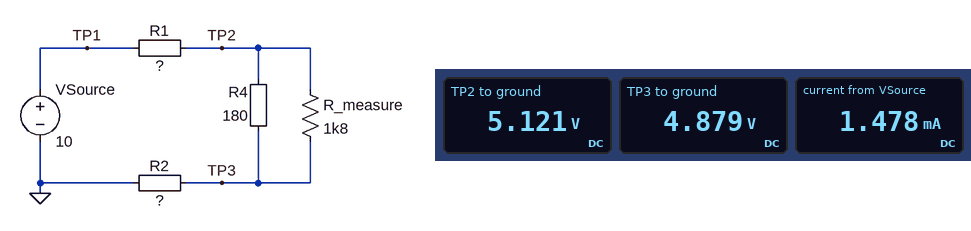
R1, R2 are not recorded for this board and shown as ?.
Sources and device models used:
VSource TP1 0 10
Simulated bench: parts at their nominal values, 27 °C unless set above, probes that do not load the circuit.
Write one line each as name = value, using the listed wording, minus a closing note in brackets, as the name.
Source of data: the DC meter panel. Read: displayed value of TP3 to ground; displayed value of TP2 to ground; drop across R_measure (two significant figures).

displayed value of TP3 to ground = 4.879 V
displayed value of TP2 to ground = 5.121 V
drop across R_measure = 240 mV
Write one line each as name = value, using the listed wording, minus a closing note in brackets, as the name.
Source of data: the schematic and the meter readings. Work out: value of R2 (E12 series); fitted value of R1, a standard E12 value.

value of R2 = 3.3 kΩ
fitted value of R1, a standard E12 value = 3.3 kΩ
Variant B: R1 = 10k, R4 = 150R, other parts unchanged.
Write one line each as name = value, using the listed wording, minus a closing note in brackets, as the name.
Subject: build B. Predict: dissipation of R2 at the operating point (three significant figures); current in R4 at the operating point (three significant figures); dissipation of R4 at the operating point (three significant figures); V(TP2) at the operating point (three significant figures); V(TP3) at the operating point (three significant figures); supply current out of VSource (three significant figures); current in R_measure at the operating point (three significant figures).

dissipation of R2 at the operating point = 1.83 mW
current in R4 at the operating point = 687 µA
dissipation of R4 at the operating point = 70.8 µW
V(TP2) at the operating point = 2.56 V
V(TP3) at the operating point = 2.46 V
supply current out of VSource = 744 µA
current in R_measure at the operating point = 57.2 µA
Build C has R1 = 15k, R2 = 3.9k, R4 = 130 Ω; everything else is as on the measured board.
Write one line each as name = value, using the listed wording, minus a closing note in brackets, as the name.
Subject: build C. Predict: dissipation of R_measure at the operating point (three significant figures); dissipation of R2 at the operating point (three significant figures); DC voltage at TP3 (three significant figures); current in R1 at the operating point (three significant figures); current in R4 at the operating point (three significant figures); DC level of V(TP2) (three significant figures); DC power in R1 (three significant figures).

dissipation of R_measure at the operating point = 2.26 µW
dissipation of R2 at the operating point = 1.08 mW
DC voltage at TP3 = 2.05 V
current in R1 at the operating point = 526 µA
current in R4 at the operating point = 490 µA
DC level of V(TP2) = 2.11 V
DC power in R1 = 4.15 mW
